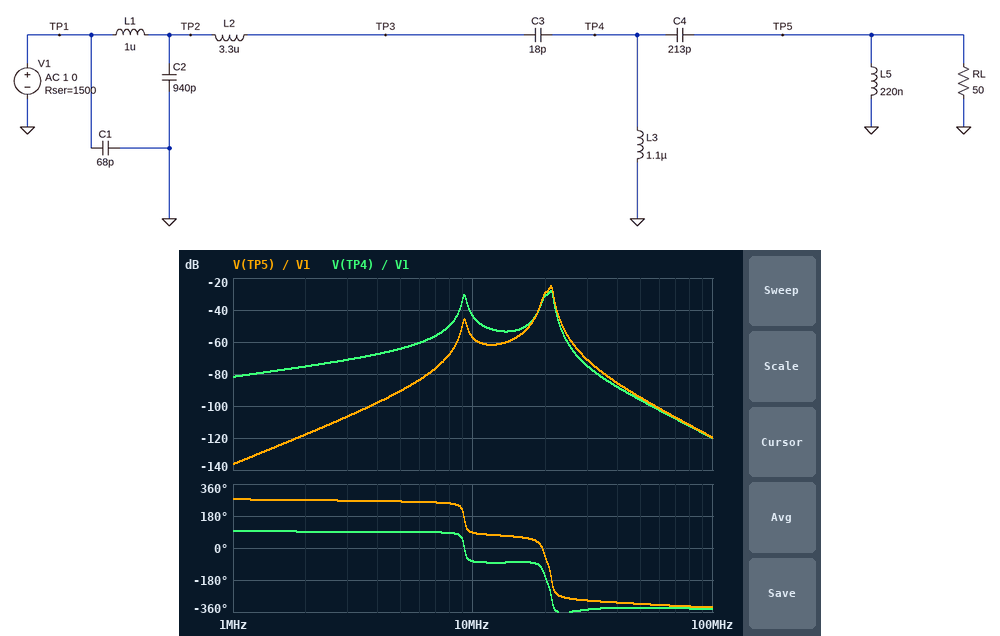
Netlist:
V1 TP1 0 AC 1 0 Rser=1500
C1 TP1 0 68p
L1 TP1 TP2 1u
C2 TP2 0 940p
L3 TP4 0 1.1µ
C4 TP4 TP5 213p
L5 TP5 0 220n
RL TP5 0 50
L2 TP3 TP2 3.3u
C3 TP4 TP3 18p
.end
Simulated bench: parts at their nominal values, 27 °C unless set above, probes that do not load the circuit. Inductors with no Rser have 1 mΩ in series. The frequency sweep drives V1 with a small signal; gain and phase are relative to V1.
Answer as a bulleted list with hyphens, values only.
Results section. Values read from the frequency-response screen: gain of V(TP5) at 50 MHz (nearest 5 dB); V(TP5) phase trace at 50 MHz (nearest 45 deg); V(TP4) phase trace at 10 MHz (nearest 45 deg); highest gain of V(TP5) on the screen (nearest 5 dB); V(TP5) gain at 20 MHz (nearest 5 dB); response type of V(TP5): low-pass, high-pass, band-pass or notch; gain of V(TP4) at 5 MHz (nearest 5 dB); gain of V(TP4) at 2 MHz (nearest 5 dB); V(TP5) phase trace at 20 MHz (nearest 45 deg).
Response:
- -95 dB
- -315 deg
- -90 deg
- -25 dB
- -30 dB
- band-pass
- -65 dB
- -75 dB
- -45 deg
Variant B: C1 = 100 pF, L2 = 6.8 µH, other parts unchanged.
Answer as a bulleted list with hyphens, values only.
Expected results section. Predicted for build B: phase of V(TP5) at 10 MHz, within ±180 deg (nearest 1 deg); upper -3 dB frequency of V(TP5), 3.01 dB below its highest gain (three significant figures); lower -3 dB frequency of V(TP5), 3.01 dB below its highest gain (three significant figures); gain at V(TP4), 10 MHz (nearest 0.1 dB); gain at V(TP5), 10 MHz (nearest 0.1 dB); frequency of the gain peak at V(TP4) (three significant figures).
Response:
- 83 deg
- 15.2 MHz
- 14.8 MHz
- -41.2 dB
- -54.6 dB
- 15.0 MHz
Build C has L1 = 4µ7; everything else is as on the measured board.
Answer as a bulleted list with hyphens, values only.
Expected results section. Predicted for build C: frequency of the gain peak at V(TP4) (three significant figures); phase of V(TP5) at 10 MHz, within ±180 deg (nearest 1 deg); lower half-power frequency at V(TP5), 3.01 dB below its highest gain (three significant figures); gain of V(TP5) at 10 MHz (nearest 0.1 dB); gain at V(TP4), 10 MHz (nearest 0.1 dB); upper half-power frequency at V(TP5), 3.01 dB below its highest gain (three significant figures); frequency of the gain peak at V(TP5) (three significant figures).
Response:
- 9.20 MHz
- -48 deg
- 9.05 MHz
- -47.8 dB
- -34.4 dB
- 9.37 MHz
- 9.21 MHz
